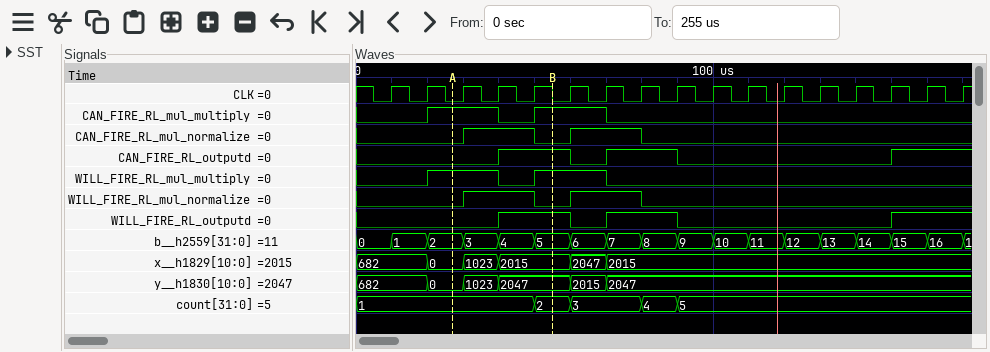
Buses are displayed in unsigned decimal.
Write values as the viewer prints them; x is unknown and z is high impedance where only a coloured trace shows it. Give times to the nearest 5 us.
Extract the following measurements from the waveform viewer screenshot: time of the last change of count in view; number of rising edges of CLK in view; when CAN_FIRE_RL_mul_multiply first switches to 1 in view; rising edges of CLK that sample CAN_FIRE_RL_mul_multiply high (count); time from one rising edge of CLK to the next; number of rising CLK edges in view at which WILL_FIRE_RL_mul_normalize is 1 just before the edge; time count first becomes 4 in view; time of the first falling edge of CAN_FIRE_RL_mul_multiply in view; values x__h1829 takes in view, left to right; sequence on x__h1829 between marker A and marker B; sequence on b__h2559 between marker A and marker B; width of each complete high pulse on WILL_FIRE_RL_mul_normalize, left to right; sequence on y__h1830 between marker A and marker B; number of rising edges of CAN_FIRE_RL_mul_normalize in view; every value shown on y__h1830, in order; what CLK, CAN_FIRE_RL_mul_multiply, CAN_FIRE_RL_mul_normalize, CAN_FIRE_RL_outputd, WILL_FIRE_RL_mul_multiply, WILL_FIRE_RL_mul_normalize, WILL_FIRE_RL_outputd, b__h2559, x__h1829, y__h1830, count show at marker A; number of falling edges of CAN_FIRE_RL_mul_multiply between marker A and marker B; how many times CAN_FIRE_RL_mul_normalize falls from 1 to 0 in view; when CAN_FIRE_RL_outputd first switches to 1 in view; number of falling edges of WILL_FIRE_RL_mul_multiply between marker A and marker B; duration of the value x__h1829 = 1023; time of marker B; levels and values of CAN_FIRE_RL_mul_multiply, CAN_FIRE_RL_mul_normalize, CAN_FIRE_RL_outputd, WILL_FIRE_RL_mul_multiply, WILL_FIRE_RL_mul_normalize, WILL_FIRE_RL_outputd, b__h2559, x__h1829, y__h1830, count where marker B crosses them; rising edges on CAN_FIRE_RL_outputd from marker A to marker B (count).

90 us
17
20 us
4
10 us
4
80 us
40 us
682, 0, 1023, 2015, 2047, 2015
0, 1023, 2015
2, 3, 4, 5
20 us, 20 us
0, 1023, 2047
2
682, 0, 1023, 2047, 2015, 2047
CLK=0, CAN_FIRE_RL_mul_multiply=1, CAN_FIRE_RL_mul_normalize=0, CAN_FIRE_RL_outputd=0, WILL_FIRE_RL_mul_multiply=1, WILL_FIRE_RL_mul_normalize=0, WILL_FIRE_RL_outputd=0, b__h2559=2, x__h1829=0, y__h1830=0, count=1
1
2
40 us
1
10 us
55 us
CAN_FIRE_RL_mul_multiply=1, CAN_FIRE_RL_mul_normalize=0, CAN_FIRE_RL_outputd=1, WILL_FIRE_RL_mul_multiply=1, WILL_FIRE_RL_mul_normalize=0, WILL_FIRE_RL_outputd=1, b__h2559=5, x__h1829=2015, y__h1830=2047, count=2
1
